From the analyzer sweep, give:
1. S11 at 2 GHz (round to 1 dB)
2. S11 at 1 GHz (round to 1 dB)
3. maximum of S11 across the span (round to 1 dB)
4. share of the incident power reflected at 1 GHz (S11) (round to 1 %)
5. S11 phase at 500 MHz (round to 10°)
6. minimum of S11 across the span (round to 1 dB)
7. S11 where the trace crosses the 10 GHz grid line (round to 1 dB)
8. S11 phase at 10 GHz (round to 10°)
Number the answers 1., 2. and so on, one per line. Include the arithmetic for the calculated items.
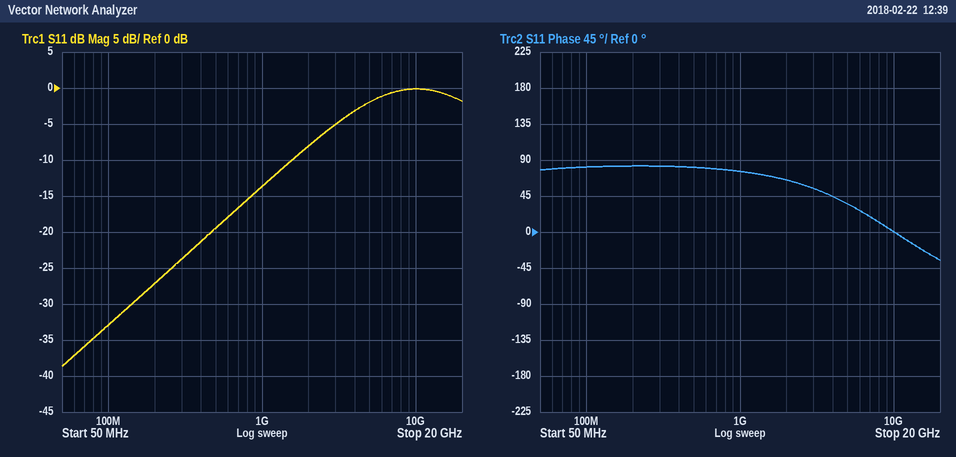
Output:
1. -8 dB
2. -14 dB
3. 0 dB
4. 10^(-14/10) ≈ 4 %
5. 80°
6. -39 dB
7. 0 dB
8. 0°
